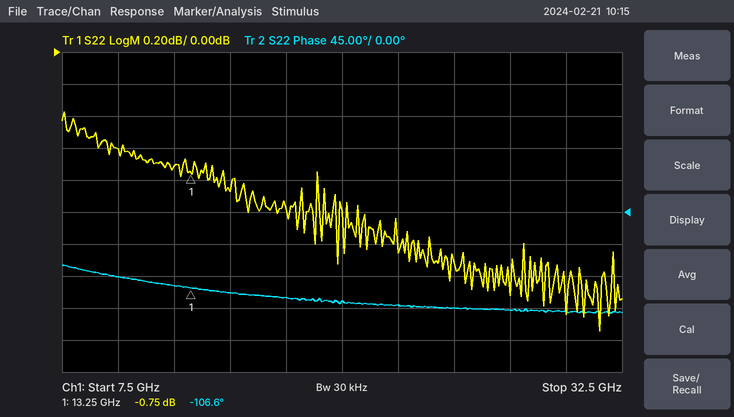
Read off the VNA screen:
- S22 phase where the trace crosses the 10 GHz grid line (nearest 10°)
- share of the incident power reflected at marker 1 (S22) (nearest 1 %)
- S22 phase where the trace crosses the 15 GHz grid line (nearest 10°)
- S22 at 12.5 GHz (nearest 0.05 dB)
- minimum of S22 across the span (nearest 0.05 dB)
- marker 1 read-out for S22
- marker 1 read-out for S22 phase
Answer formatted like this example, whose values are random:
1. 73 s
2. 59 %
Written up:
1. -90°
2. 84 %
3. -110°
4. -0.70 dB
5. -1.75 dB
6. -0.75 dB
7. -106.6°
